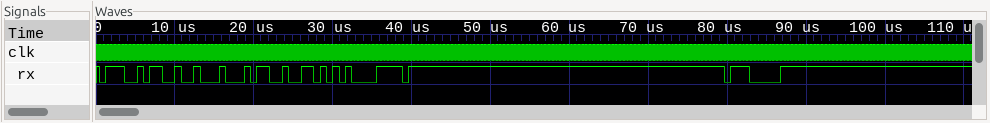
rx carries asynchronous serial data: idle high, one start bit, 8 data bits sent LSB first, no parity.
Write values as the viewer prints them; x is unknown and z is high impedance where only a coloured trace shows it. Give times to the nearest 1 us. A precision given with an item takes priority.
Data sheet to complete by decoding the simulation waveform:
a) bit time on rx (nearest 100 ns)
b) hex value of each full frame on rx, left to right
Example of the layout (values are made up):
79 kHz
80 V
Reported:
800 ns
A7, 12, 34, 56, 78, 07
